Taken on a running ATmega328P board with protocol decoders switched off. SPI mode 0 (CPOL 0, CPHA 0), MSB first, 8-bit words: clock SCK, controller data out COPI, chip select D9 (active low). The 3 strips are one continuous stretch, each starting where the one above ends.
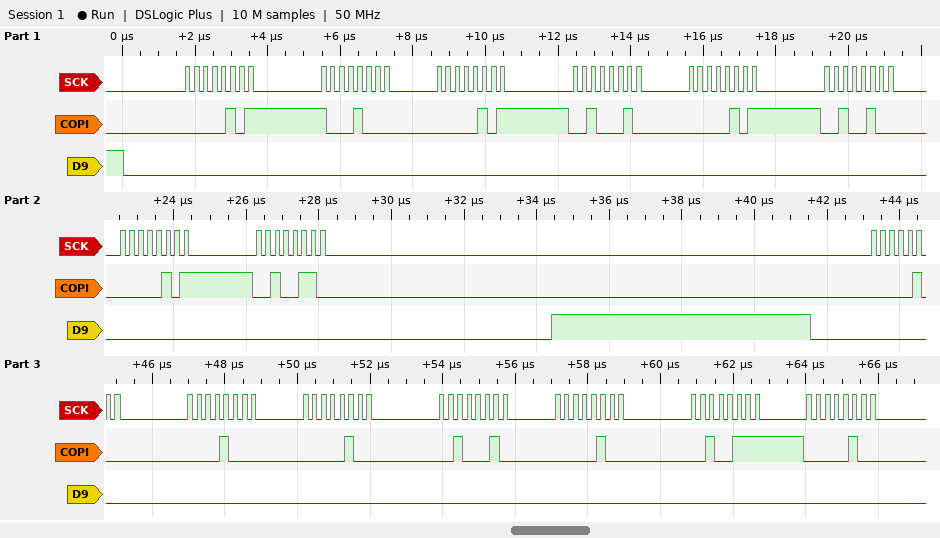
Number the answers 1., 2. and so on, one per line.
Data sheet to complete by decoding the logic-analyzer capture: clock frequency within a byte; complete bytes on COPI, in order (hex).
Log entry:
1. 4 MHz
2. 05 88 05 22 05 24 05 26 04 08 04 22 04 27 04
